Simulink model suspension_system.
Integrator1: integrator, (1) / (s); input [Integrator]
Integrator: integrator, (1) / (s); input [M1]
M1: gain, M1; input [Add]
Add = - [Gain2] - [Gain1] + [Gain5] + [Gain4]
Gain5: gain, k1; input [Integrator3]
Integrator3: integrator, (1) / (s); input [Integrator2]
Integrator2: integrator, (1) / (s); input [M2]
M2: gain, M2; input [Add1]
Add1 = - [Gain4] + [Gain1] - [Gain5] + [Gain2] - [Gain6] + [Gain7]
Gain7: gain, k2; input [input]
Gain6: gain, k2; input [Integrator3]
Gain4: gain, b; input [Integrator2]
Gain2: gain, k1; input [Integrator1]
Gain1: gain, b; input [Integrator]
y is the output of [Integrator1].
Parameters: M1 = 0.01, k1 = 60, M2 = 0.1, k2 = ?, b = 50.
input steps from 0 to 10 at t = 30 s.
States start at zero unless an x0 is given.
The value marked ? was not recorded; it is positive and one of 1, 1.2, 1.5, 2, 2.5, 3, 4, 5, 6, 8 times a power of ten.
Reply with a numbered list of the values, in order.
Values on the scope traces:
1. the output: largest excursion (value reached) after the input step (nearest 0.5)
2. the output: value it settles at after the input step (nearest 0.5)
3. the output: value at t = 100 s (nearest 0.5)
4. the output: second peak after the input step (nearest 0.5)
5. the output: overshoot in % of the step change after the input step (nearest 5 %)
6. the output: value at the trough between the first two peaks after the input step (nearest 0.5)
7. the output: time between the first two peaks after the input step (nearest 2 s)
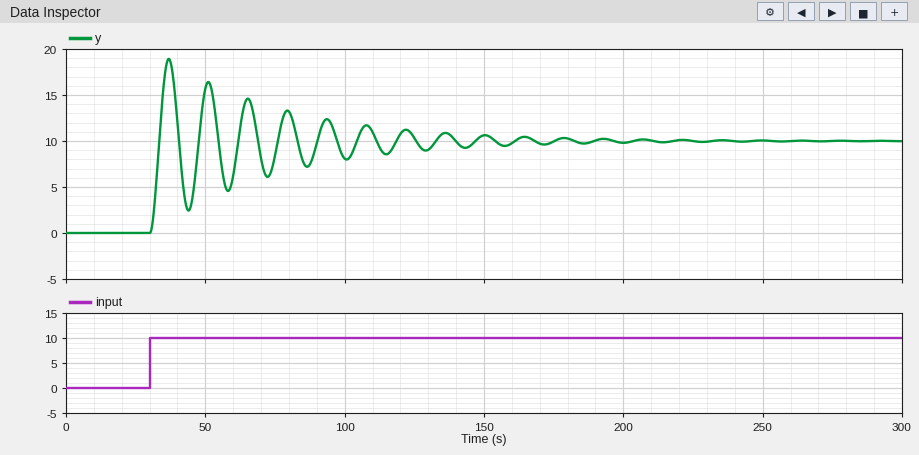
1. 19.0
2. 10.0
3. 8.0
4. 16.5
5. 90 %
6. 2.5
7. 14 s
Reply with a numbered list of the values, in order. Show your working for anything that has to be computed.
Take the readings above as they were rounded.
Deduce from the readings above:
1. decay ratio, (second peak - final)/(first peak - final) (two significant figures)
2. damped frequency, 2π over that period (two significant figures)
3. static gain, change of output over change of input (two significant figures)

1. (16.5 - 10) / (19 - 10) = 0.72
2. 2π / 14 = 0.45 rad/s
3. (10 - 0) / (10 - 0) = 1.0
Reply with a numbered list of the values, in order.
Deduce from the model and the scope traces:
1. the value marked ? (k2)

1. 30
